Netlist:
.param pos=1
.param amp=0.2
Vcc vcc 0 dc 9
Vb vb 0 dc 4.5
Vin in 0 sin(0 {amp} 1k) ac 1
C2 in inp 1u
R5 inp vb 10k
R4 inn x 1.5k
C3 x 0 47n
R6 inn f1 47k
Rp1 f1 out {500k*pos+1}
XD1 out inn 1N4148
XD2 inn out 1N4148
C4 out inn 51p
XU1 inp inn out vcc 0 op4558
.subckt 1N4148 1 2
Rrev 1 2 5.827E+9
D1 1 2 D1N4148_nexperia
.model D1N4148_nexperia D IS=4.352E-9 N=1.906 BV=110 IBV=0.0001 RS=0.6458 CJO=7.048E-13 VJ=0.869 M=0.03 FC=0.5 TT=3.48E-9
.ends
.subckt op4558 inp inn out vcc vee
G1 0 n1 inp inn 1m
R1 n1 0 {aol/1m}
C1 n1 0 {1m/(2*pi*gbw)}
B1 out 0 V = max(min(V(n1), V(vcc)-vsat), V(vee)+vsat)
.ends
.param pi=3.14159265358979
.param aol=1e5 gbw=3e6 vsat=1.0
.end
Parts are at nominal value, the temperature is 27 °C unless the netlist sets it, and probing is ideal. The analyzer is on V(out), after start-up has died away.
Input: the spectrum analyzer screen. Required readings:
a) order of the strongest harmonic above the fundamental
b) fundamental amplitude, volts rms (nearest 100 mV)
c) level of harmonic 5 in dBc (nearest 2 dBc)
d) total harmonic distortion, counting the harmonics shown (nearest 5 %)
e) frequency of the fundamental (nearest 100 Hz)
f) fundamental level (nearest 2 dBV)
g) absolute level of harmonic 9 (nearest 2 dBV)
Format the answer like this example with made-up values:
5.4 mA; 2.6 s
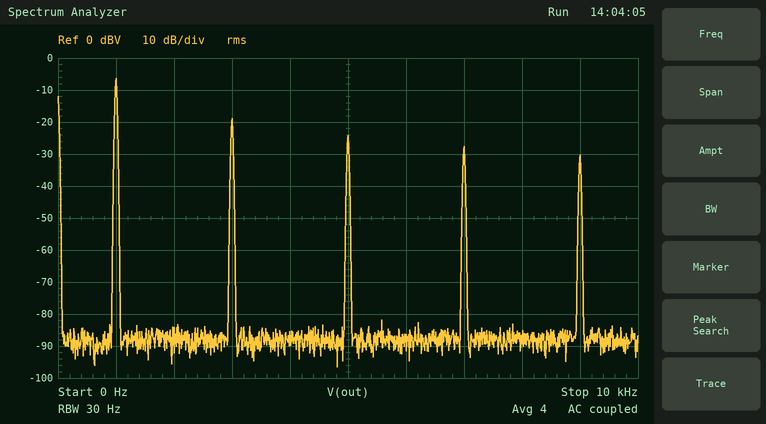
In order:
3; 500 mV; -18 dBc; 30 %; 1.0 kHz; -6 dBV; -30 dBV
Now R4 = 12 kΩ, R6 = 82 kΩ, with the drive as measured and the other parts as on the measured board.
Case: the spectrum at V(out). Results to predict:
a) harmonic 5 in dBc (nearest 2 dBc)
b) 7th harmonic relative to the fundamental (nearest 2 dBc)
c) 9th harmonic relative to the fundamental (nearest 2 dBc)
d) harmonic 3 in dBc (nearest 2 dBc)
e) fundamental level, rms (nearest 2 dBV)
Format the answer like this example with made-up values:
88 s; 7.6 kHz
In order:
-20 dBc; -24 dBc; -26 dBc; -14 dBc; -6 dBV
